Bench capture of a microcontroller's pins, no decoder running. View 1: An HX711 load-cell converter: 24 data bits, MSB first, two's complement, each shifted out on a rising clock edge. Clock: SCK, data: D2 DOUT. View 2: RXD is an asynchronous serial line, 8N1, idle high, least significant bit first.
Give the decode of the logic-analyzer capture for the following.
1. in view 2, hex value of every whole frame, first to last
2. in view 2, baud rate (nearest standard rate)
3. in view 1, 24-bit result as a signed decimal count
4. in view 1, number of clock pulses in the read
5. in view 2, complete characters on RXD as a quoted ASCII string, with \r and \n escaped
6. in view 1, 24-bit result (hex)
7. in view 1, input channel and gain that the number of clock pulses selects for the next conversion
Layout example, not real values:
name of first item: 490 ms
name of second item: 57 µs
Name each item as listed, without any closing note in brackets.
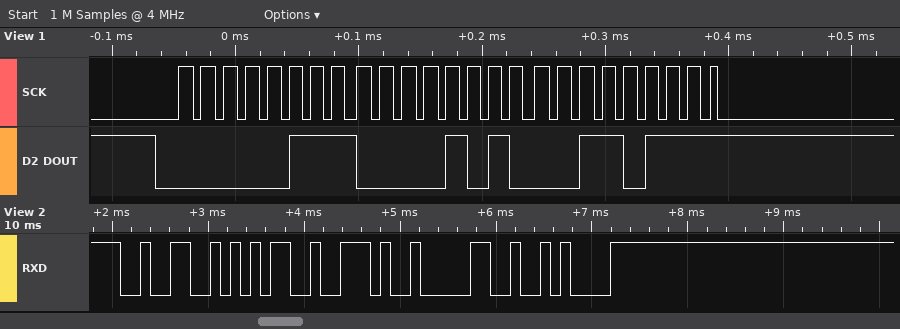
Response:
in view 2, hex value of every whole frame, first to last: 0x32 0x35 0x2E 0x30 0x0A
in view 2, baud rate: 9600 baud
in view 1, 24-bit result as a signed decimal count: 461367
in view 1, number of clock pulses in the read: 25
in view 2, complete characters on RXD as a quoted ASCII string, with \r and \n escaped: "25.0\n"
in view 1, 24-bit result: 0x070A37
in view 1, input channel and gain that the number of clock pulses selects for the next conversion: channel A, gain 128
